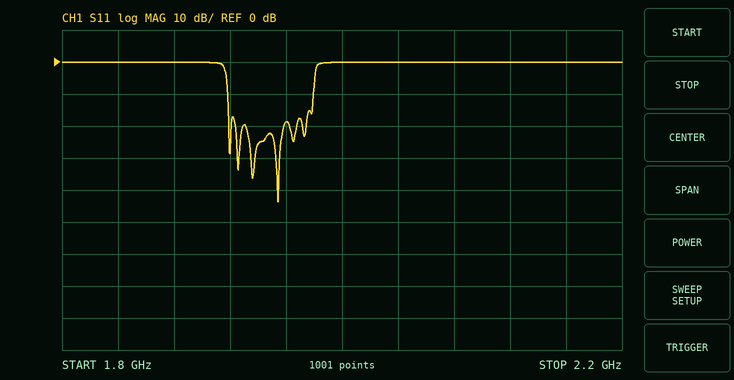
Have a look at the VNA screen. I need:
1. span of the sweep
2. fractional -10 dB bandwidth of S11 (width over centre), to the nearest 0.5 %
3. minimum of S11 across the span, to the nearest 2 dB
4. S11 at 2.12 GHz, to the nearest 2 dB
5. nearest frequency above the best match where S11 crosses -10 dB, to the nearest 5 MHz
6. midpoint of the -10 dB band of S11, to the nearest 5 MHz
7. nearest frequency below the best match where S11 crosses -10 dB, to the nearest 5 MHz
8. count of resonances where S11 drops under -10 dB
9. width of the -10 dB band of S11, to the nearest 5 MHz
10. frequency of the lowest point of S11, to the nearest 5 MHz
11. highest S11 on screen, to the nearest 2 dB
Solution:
400 MHz
3.0 %
-44 dB
0 dB
1.980 GHz
1.950 GHz
1.920 GHz
6
60 MHz
1.955 GHz
0 dB
